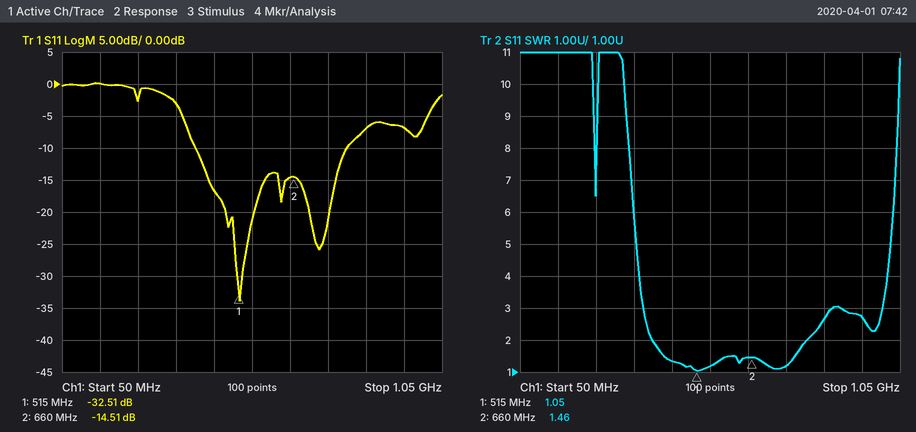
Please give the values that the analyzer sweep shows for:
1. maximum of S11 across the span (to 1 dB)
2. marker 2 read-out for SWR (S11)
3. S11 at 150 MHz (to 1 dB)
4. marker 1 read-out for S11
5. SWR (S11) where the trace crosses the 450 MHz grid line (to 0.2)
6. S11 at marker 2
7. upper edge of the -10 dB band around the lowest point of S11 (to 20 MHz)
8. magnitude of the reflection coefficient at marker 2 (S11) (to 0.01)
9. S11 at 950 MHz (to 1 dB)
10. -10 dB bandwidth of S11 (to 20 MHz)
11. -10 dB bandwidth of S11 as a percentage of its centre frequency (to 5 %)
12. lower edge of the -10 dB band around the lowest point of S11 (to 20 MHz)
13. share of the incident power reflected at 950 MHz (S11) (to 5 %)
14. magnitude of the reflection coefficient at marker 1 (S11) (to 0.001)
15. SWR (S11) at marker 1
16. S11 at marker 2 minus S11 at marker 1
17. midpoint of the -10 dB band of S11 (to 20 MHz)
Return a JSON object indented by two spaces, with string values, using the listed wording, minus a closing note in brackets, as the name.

{
  "maximum of S11 across the span": "0 dB",
  "marker 2 read-out for SWR": "1.46",
  "S11 at 150 MHz": "0 dB",
  "marker 1 read-out for S11": "-32.51 dB",
  "SWR (S11) where the trace crosses the 450 MHz grid line": "1.4",
  "S11 at marker 2": "-14.51 dB",
  "upper edge of the -10 dB band around the lowest point of S11": "800 MHz",
  "magnitude of the reflection coefficient at marker 2 (S11)": "0.19",
  "S11 at 950 MHz": "-7 dB",
  "-10 dB bandwidth of S11": "400 MHz",
  "-10 dB bandwidth of S11 as a percentage of its centre frequency": "65 %",
  "lower edge of the -10 dB band around the lowest point of S11": "400 MHz",
  "share of the incident power reflected at 950 MHz (S11)": "20 %",
  "magnitude of the reflection coefficient at marker 1 (S11)": "0.024",
  "SWR (S11) at marker 1": "1.05",
  "S11 at marker 2 minus S11 at marker 1": "18.00 dB",
  "midpoint of the -10 dB band of S11": "600 MHz"
}
